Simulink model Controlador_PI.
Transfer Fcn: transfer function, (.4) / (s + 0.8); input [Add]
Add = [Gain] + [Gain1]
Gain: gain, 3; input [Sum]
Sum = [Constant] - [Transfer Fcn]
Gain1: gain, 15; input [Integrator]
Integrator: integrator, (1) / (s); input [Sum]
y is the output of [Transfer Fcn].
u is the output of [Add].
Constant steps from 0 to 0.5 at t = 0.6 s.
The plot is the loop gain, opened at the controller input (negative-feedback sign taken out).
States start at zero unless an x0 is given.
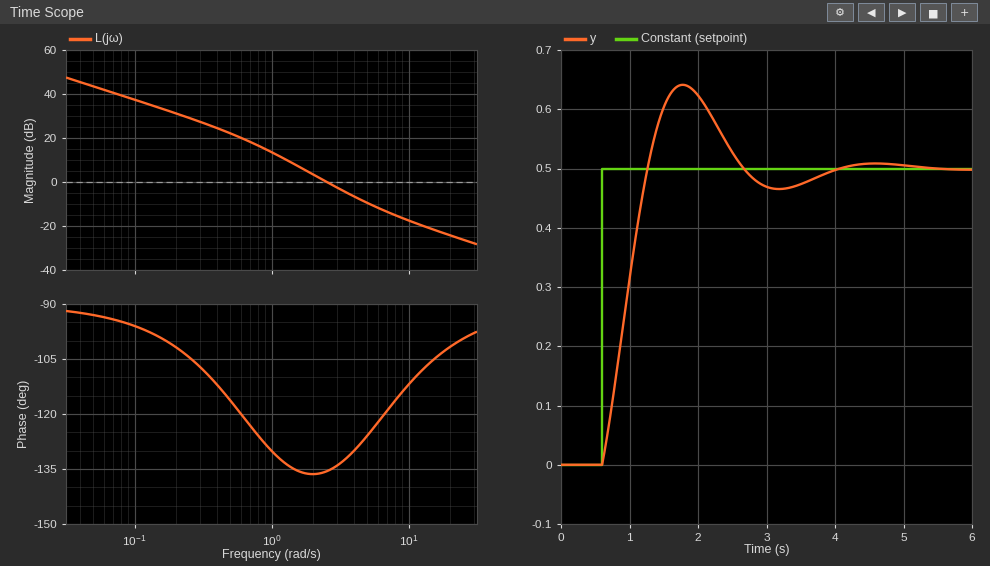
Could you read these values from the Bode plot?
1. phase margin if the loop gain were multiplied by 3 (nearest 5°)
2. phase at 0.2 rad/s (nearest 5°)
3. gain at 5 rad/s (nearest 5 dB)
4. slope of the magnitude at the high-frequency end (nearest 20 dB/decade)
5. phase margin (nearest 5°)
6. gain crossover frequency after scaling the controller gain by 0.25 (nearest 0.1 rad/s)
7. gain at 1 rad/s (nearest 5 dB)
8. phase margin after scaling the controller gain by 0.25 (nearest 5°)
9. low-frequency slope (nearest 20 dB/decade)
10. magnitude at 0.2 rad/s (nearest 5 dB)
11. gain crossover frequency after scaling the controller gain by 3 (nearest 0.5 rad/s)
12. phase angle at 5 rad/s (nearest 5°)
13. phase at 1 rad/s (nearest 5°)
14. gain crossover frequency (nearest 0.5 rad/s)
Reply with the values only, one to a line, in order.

55°
-100°
-10 dB
-20 dB/decade
45°
1.1 rad/s
15 dB
50°
-20 dB/decade
30 dB
5.0 rad/s
-125°
-130°
2.5 rad/s
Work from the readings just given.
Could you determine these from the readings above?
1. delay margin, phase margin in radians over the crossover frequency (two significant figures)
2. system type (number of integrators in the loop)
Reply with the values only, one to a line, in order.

0.31 s
1
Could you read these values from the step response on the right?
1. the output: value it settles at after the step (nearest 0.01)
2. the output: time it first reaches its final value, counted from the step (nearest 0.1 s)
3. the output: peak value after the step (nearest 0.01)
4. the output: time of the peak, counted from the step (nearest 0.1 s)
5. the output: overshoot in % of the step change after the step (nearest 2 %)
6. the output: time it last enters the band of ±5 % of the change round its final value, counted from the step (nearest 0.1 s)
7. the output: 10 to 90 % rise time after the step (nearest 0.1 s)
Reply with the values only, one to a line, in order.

0.50
0.7 s
0.64
1.2 s
28 %
2.9 s
0.5 s
